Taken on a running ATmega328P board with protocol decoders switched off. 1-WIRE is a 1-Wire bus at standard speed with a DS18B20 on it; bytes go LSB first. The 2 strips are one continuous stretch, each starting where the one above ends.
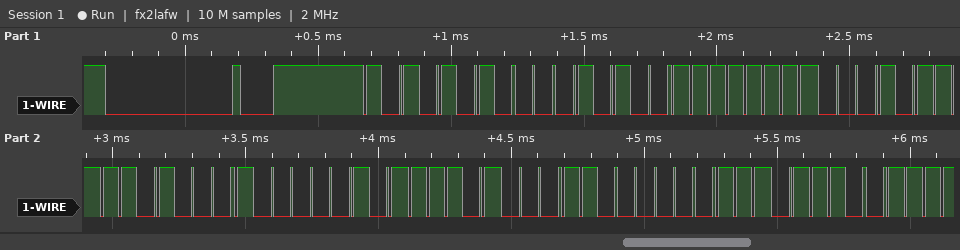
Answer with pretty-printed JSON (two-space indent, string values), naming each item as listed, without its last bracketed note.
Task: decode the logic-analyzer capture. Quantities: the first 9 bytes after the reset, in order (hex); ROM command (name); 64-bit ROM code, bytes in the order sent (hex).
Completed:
{
  "the first 9 bytes after the reset, in order": "55 28 FF E8 8B A0 17 03 77",
  "ROM command": "Match ROM",
  "64-bit ROM code, bytes in the order sent": "28 FF E8 8B A0 17 03 77"
}
